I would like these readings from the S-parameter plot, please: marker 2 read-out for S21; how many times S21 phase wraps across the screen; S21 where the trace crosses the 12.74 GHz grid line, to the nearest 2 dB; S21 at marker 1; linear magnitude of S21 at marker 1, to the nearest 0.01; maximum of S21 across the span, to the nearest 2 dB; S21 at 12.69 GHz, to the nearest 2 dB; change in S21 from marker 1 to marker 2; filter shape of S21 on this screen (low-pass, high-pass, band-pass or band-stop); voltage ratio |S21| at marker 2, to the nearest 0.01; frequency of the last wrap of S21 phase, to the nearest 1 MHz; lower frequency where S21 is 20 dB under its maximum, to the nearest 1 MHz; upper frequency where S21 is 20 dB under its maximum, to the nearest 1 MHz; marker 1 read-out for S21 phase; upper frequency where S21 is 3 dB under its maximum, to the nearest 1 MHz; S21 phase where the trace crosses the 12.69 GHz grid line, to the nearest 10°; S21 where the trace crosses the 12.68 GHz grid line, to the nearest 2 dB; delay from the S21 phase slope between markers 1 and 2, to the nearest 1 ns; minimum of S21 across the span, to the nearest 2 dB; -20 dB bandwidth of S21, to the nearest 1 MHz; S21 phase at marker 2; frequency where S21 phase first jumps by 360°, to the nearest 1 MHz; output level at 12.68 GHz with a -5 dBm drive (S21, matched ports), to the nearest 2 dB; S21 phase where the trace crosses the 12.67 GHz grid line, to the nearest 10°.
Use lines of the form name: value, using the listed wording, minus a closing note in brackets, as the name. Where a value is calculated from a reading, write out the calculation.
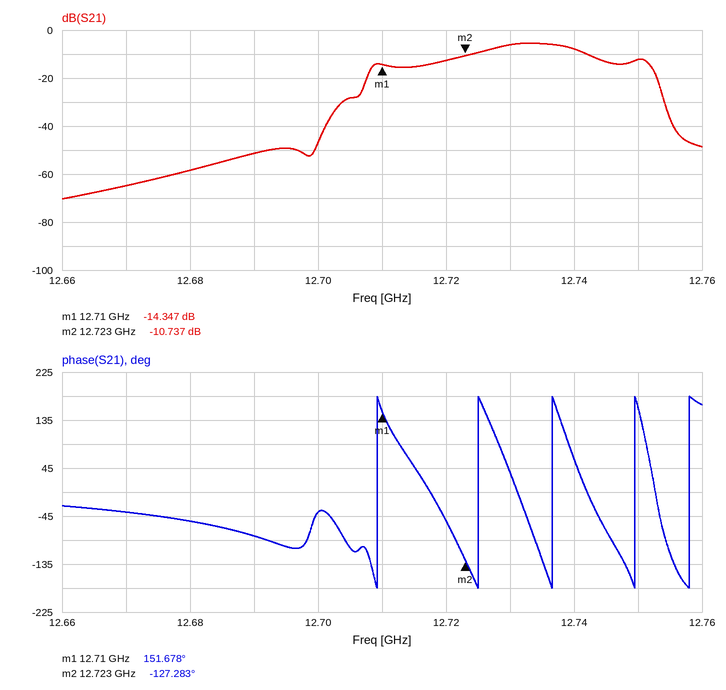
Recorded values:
marker 2 read-out for S21: -10.737 dB
how many times S21 phase wraps across the screen: 5
S21 where the trace crosses the 12.74 GHz grid line, to the nearest 2 dB: -8 dB
S21 at marker 1: -14.347 dB
linear magnitude of S21 at marker 1, to the nearest 0.01: 10^(-14.347/20) ≈ 0.19
maximum of S21 across the span, to the nearest 2 dB: -6 dB
S21 at 12.69 GHz, to the nearest 2 dB: -52 dB
change in S21 from marker 1 to marker 2: -10.737 − (-14.347) = 3.610 dB
filter shape of S21 on this screen: band-pass
voltage ratio |S21| at marker 2, to the nearest 0.01: 10^(-10.737/20) ≈ 0.29
frequency of the last wrap of S21 phase, to the nearest 1 MHz: 12.758 GHz
lower frequency where S21 is 20 dB under its maximum, to the nearest 1 MHz: 12.707 GHz
upper frequency where S21 is 20 dB under its maximum, to the nearest 1 MHz: 12.754 GHz
marker 1 read-out for S21 phase: 151.678°
upper frequency where S21 is 3 dB under its maximum, to the nearest 1 MHz: 12.741 GHz
S21 phase where the trace crosses the 12.69 GHz grid line, to the nearest 10°: -80°
S21 where the trace crosses the 12.68 GHz grid line, to the nearest 2 dB: -58 dB
delay from the S21 phase slope between markers 1 and 2, to the nearest 1 ns: −(-127.283° − (151.678°))/(360° × 13 MHz) ≈ 60 ns
minimum of S21 across the span, to the nearest 2 dB: -70 dB
-20 dB bandwidth of S21, to the nearest 1 MHz: 12.754 GHz − 12.707 GHz = 47 MHz
S21 phase at marker 2: -127.283°
frequency where S21 phase first jumps by 360°, to the nearest 1 MHz: 12.709 GHz
output level at 12.68 GHz with a -5 dBm drive (S21, matched ports), to the nearest 2 dB: -5 dBm + (-58 dB) = -64 dBm
S21 phase where the trace crosses the 12.67 GHz grid line, to the nearest 10°: -40°
